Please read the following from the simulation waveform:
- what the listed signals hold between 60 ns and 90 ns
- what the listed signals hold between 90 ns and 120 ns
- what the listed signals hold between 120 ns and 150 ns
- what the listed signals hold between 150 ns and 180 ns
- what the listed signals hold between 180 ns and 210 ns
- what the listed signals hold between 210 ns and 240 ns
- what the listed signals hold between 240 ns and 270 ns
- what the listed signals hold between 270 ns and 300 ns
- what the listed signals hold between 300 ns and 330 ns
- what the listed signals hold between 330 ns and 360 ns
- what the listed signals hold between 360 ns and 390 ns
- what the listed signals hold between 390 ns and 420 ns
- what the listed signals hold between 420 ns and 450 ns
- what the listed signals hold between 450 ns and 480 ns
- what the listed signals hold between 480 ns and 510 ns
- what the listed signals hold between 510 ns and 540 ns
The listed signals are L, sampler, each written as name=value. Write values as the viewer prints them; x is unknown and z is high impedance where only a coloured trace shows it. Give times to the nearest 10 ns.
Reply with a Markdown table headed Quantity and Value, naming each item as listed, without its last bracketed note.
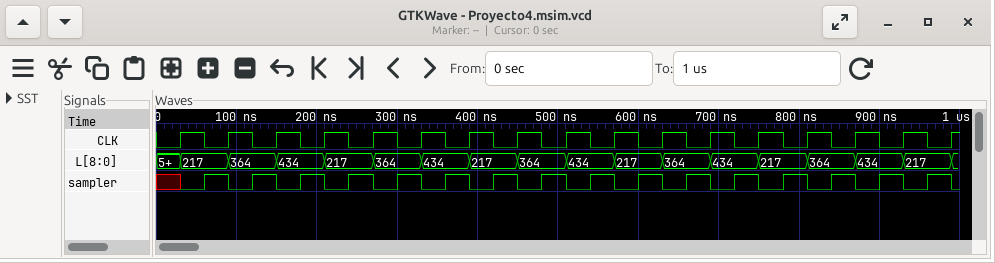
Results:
| Quantity | Value |
|---|---|
| what the listed signals hold between 60 ns and 90 ns | L=217, sampler=1 |
| what the listed signals hold between 90 ns and 120 ns | L=364, sampler=0 |
| what the listed signals hold between 120 ns and 150 ns | L=364, sampler=1 |
| what the listed signals hold between 150 ns and 180 ns | L=434, sampler=0 |
| what the listed signals hold between 180 ns and 210 ns | L=434, sampler=1 |
| what the listed signals hold between 210 ns and 240 ns | L=217, sampler=0 |
| what the listed signals hold between 240 ns and 270 ns | L=217, sampler=1 |
| what the listed signals hold between 270 ns and 300 ns | L=364, sampler=0 |
| what the listed signals hold between 300 ns and 330 ns | L=364, sampler=1 |
| what the listed signals hold between 330 ns and 360 ns | L=434, sampler=0 |
| what the listed signals hold between 360 ns and 390 ns | L=434, sampler=1 |
| what the listed signals hold between 390 ns and 420 ns | L=217, sampler=0 |
| what the listed signals hold between 420 ns and 450 ns | L=217, sampler=1 |
| what the listed signals hold between 450 ns and 480 ns | L=364, sampler=0 |
| what the listed signals hold between 480 ns and 510 ns | L=364, sampler=1 |
| what the listed signals hold between 510 ns and 540 ns | L=434, sampler=0 |
